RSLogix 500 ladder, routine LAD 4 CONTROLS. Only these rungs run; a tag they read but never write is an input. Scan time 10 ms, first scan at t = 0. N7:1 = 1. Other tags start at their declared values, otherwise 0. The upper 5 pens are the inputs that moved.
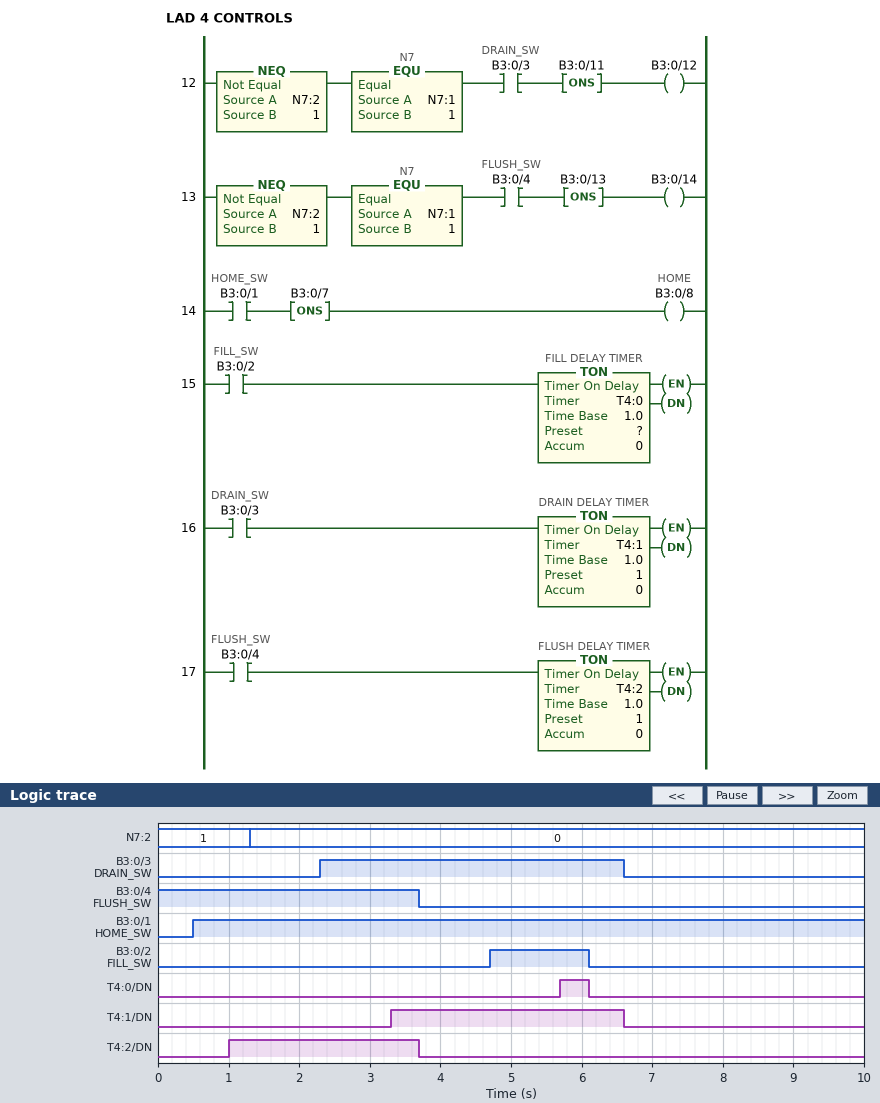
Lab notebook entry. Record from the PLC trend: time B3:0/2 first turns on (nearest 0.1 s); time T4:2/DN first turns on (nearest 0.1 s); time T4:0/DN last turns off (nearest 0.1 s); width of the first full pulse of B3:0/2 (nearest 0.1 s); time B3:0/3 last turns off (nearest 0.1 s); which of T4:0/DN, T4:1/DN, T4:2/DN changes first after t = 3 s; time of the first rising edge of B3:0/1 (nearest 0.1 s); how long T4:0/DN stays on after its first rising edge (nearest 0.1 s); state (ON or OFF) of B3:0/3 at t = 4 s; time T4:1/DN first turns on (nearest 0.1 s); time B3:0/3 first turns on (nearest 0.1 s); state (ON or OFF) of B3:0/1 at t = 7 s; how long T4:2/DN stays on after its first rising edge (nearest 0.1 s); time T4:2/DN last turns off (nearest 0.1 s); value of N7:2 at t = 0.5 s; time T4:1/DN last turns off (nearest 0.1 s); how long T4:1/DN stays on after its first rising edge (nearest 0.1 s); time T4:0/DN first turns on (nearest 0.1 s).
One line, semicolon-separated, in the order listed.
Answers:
4.7 s; 1.0 s; 6.1 s; 1.4 s; 6.6 s; T4:1/DN; 0.5 s; 0.4 s; ON; 3.3 s; 2.3 s; ON; 2.7 s; 3.7 s; 1; 6.6 s; 3.3 s; 5.7 s
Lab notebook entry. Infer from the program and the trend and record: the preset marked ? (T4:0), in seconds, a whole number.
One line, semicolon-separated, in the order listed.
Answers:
1 s
